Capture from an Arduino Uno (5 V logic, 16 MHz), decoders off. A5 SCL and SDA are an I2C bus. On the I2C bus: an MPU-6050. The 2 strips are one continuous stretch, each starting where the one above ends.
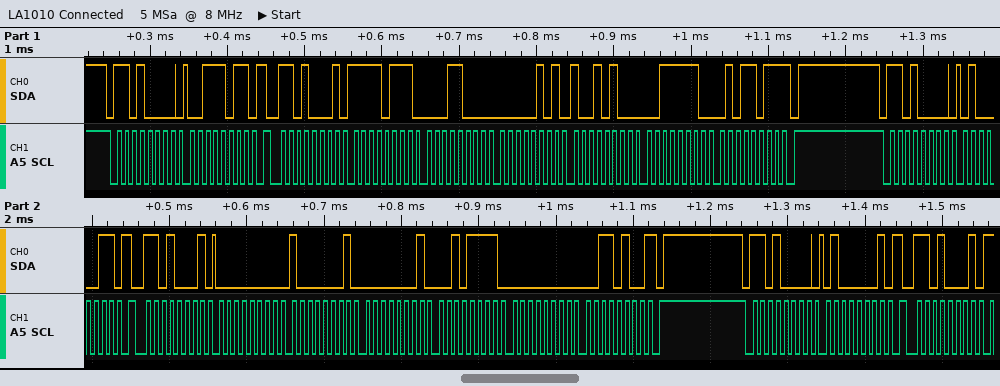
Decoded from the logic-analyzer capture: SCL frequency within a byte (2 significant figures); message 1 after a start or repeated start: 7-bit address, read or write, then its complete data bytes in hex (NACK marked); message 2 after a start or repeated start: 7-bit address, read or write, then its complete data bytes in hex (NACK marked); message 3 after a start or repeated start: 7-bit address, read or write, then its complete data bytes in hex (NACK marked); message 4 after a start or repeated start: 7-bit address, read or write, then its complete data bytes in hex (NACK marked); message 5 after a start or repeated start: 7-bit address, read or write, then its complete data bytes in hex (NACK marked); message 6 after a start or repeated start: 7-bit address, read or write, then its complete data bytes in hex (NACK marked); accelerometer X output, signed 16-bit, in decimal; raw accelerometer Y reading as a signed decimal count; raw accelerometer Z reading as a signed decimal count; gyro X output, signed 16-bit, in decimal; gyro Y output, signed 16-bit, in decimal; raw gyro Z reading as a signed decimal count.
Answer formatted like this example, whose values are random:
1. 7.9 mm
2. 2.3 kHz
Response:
1. 100 kHz
2. 0x68 write: 3B
3. 0x68 read: F7 18 05 94 3E 5B NACK
4. 0x68 write: 43
5. 0x68 read: 00 81 01 2F 00 34 NACK
6. 0x68 write: 41
7. 0x68 read
8. -2280
9. 1428
10. 15963
11. 129
12. 303
13. 52
